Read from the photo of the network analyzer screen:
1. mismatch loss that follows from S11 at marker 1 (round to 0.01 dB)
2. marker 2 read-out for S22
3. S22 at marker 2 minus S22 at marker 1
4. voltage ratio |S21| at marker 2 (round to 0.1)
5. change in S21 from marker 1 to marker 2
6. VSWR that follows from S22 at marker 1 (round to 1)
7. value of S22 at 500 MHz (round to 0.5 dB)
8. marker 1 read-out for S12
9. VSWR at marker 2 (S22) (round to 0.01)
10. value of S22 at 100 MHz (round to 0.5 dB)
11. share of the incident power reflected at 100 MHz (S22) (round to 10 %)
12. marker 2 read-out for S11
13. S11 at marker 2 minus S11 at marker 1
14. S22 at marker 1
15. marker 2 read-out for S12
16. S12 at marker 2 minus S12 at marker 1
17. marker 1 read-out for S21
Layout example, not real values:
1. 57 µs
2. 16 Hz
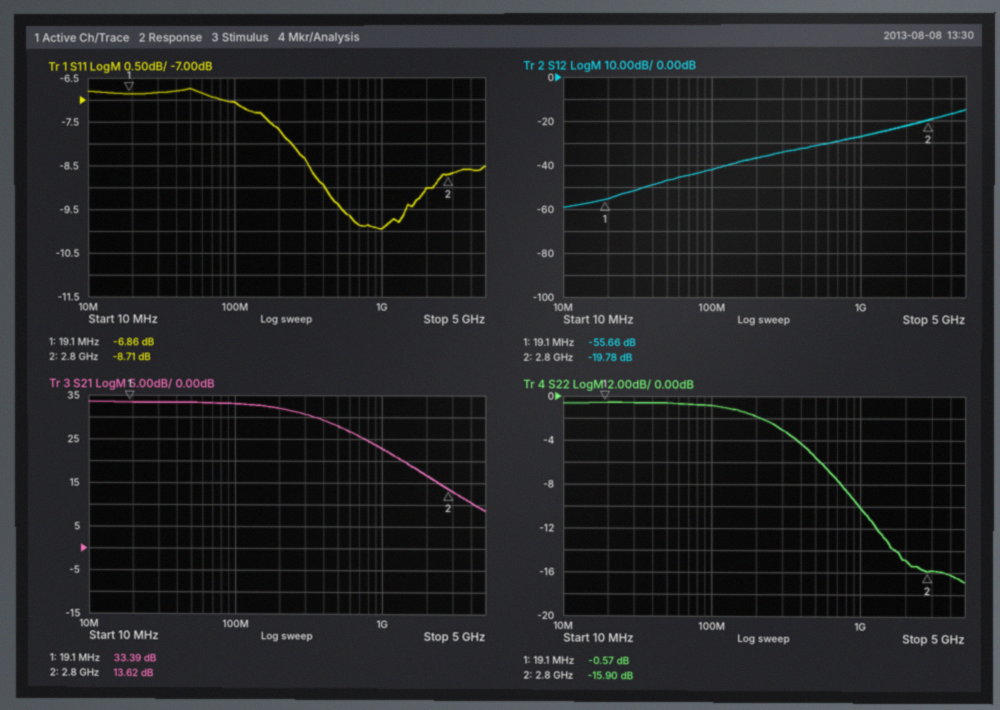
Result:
1. 1.00 dB
2. -15.90 dB
3. -15.33 dB
4. 4.8
5. -19.77 dB
6. 30
7. -5.5 dB
8. -55.66 dB
9. 1.38
10. -1.0 dB
11. 80 %
12. -8.71 dB
13. -1.85 dB
14. -0.57 dB
15. -19.78 dB
16. 35.88 dB
17. 33.39 dB
